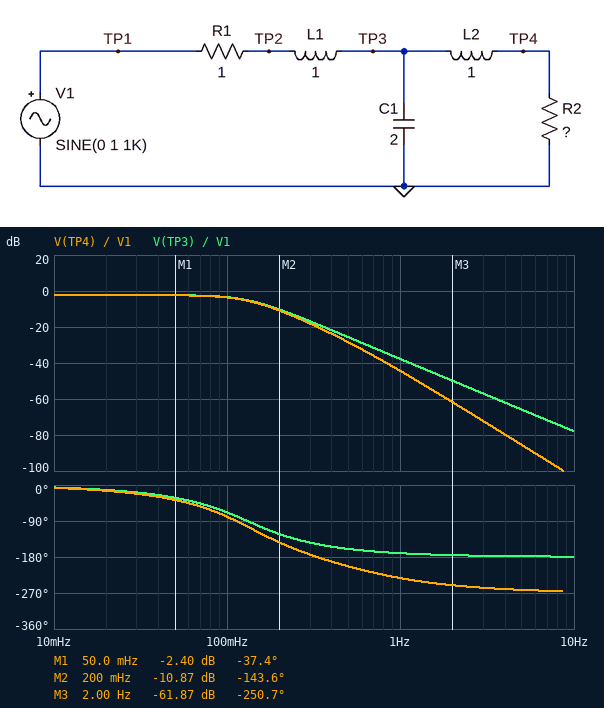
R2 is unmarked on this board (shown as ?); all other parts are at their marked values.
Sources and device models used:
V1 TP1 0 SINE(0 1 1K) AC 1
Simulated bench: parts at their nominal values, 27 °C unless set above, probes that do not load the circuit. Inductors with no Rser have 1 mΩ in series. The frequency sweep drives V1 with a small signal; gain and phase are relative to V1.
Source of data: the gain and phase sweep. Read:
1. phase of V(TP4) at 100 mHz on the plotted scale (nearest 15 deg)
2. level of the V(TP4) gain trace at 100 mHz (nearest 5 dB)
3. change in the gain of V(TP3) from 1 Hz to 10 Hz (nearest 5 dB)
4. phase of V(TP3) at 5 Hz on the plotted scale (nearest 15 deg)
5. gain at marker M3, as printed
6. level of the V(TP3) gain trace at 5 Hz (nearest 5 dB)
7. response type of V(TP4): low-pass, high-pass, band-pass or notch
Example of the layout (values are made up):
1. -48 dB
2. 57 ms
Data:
1. -75 deg
2. -5 dB
3. -40 dB
4. -180 deg
5. -61.87 dB
6. -65 dB
7. low-pass
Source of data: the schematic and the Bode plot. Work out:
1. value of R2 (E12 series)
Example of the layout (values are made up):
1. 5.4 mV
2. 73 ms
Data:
1. 3.3 Ω
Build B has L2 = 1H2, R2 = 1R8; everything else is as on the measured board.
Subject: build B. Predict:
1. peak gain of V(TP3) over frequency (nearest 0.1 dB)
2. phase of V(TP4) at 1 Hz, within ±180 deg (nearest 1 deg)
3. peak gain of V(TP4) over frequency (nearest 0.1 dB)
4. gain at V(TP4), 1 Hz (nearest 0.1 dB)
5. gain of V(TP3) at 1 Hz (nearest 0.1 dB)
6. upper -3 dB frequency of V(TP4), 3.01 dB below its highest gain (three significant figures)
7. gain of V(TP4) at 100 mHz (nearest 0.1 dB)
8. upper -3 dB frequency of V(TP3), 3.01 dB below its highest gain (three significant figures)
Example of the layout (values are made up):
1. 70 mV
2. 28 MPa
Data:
1. -3.7 dB
2. 113 deg
3. -3.8 dB
4. -50.5 dB
5. -37.9 dB
6. 141 mHz
7. -4.7 dB
8. 159 mHz
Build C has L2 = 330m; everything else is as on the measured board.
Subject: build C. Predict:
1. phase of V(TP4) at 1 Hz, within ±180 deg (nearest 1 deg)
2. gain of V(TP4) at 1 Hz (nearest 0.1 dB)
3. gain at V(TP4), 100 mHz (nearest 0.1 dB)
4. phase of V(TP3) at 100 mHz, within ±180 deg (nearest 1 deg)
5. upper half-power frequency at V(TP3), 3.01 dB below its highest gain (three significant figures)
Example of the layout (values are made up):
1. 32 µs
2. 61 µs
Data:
1. 158 deg
2. -39.3 dB
3. -3.7 dB
4. -70 deg
5. 129 mHz
